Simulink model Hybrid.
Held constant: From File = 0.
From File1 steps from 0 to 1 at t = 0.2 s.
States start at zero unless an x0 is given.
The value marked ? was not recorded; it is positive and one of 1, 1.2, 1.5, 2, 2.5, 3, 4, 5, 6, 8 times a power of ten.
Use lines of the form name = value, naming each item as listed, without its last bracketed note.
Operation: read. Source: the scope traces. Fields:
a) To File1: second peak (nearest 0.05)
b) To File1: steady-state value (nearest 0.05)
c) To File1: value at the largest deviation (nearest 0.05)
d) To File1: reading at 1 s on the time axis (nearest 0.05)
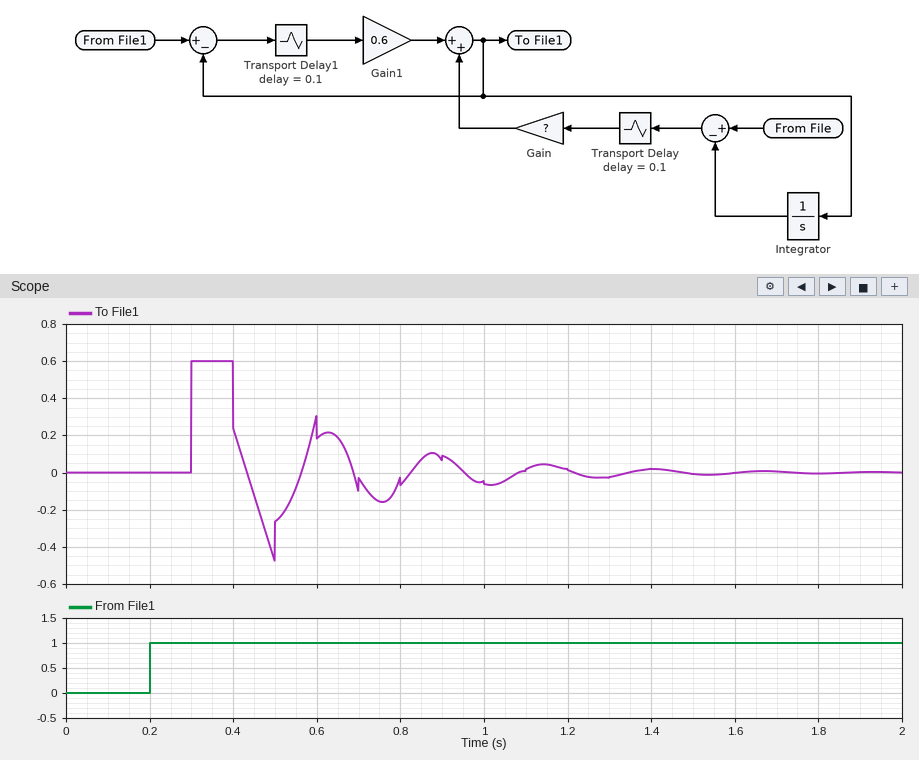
To File1: second peak = 0.30
To File1: steady-state value = 0.00
To File1: value at the largest deviation = 0.60
To File1: reading at 1 s on the time axis = -0.05
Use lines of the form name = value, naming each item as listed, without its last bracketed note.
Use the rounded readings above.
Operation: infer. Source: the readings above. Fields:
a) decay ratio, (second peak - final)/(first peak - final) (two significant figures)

decay ratio, (second peak - final)/(first peak - final) = 0.50
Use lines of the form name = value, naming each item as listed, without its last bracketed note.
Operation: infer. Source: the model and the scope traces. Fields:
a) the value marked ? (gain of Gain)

the value marked ? = 12
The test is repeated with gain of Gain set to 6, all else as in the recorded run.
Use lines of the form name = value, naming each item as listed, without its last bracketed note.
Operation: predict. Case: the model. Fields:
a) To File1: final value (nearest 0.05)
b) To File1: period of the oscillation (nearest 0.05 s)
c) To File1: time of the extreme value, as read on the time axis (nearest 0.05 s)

To File1: final value = 0.00
To File1: period of the oscillation = 0.25 s
To File1: time of the extreme value, as read on the time axis = 0.30 s
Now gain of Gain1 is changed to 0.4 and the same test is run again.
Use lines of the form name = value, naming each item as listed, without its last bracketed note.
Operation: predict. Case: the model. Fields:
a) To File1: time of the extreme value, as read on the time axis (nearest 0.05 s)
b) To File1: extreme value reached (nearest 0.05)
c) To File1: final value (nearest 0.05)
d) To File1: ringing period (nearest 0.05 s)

To File1: time of the extreme value, as read on the time axis = 0.30 s
To File1: extreme value reached = 0.40
To File1: final value = 0.00
To File1: ringing period = 0.30 s
